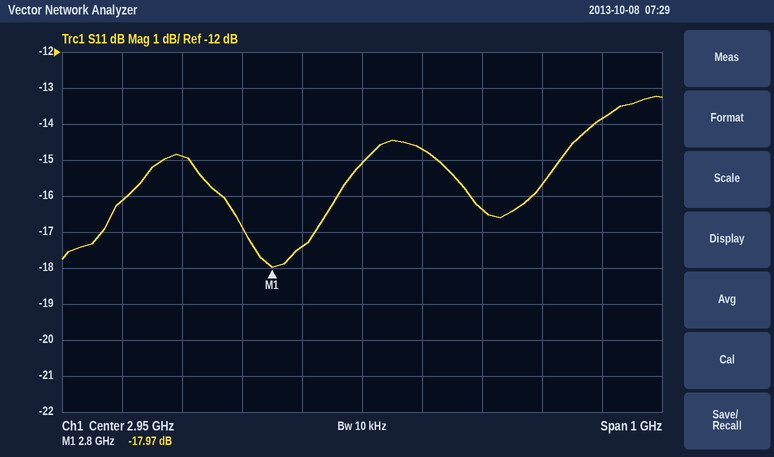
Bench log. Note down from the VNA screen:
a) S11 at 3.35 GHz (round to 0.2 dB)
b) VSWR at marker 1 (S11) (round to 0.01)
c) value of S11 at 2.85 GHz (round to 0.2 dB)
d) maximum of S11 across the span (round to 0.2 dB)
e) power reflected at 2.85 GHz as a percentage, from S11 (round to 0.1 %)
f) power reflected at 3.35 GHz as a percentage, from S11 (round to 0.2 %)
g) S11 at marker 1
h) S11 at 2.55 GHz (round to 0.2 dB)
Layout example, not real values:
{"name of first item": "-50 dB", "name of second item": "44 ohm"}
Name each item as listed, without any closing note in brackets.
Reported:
{"S11 at 3.35 GHz": "-13.8 dB", "VSWR at marker 1 (S11)": "1.29", "value of S11 at 2.85 GHz": "-17.4 dB", "maximum of S11 across the span": "-13.2 dB", "power reflected at 2.85 GHz as a percentage, from S11": "1.8 %", "power reflected at 3.35 GHz as a percentage, from S11": "4.2 %", "S11 at marker 1": "-17.97 dB", "S11 at 2.55 GHz": "-16.2 dB"}
